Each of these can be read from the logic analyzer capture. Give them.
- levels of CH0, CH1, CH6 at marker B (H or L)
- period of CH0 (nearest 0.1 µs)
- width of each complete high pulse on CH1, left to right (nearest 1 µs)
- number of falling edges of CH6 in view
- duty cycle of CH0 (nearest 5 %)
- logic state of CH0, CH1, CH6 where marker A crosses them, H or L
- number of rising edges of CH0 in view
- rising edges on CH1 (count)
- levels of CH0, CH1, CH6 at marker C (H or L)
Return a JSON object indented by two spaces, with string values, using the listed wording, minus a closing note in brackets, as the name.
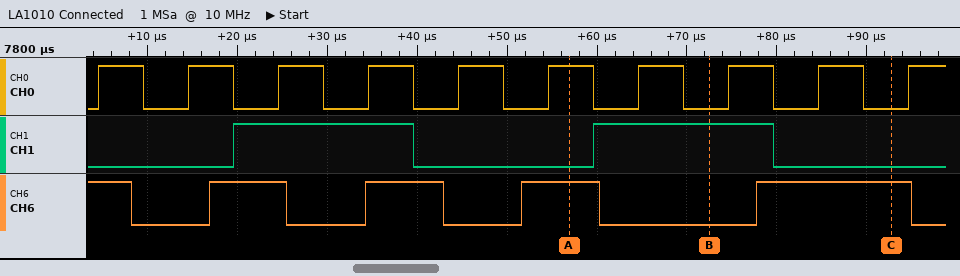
{
  "levels of CH0, CH1, CH6 at marker B": "CH0=L, CH1=H, CH6=L",
  "period of CH0": "10 µs",
  "width of each complete high pulse on CH1, left to right": "20 µs, 20 µs",
  "number of falling edges of CH6 in view": "5",
  "duty cycle of CH0": "50 %",
  "logic state of CH0, CH1, CH6 where marker A crosses them, H or L": "CH0=H, CH1=L, CH6=H",
  "number of rising edges of CH0 in view": "10",
  "rising edges on CH1": "2",
  "levels of CH0, CH1, CH6 at marker C": "CH0=L, CH1=L, CH6=H"
}
